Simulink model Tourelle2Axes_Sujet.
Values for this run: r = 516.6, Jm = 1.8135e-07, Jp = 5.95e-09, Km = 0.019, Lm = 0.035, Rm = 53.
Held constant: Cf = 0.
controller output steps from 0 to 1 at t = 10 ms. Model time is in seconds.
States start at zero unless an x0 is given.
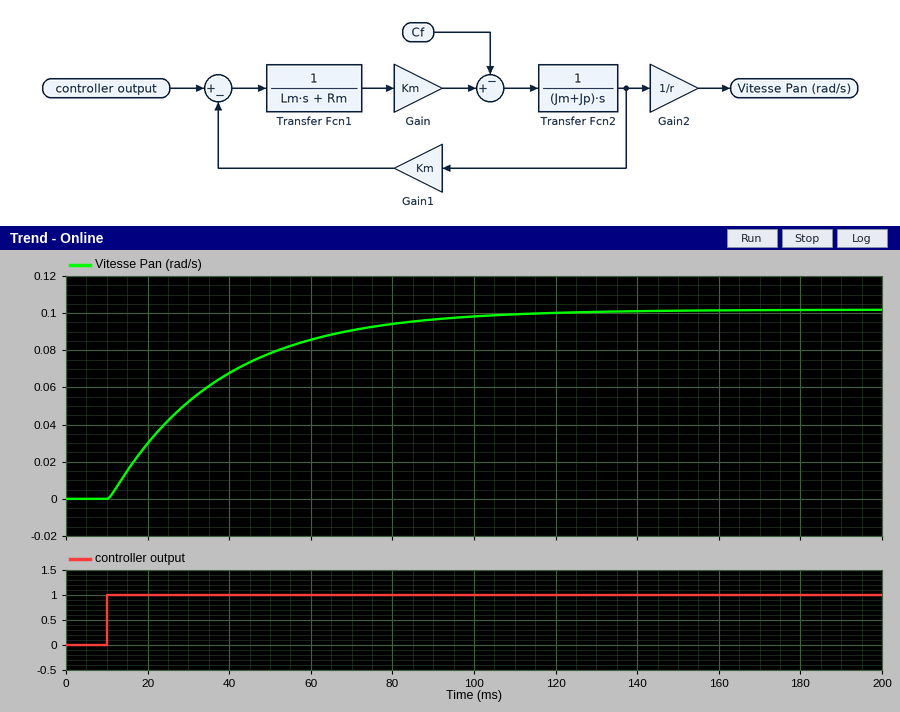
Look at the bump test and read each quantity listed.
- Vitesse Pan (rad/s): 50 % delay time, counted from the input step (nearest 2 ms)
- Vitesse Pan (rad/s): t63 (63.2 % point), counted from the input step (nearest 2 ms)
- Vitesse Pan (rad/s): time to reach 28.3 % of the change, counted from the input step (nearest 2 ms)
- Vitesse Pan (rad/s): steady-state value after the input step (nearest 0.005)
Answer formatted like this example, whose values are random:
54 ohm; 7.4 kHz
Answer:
20 ms; 28 ms; 10 ms; 0.100
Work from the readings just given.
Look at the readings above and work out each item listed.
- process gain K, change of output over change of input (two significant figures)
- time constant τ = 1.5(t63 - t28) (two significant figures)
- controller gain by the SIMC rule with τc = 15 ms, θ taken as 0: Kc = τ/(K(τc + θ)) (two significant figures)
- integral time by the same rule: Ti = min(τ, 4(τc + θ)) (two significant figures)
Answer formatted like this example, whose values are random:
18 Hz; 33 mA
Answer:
0.10; 27 ms; 18; 27 ms
